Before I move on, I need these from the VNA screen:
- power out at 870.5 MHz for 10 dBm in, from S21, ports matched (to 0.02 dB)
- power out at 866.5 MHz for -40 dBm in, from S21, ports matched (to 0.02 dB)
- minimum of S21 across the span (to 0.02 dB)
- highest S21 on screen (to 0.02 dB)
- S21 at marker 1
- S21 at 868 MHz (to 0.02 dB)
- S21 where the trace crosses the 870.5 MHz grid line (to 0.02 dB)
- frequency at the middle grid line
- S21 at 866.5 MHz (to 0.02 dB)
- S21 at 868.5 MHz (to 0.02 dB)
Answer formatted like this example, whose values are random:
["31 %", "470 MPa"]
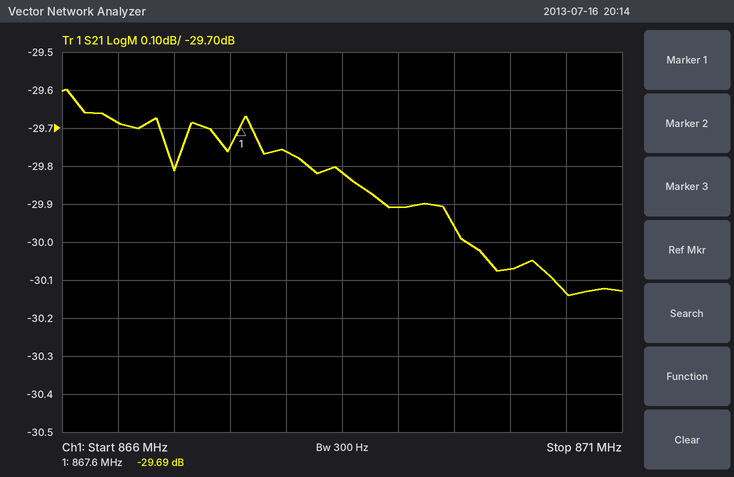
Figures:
["-20.14 dBm", "-69.68 dBm", "-30.14 dB", "-29.60 dB", "-29.69 dB", "-29.76 dB", "-30.14 dB", "868.5 MHz", "-29.68 dB", "-29.82 dB"]
